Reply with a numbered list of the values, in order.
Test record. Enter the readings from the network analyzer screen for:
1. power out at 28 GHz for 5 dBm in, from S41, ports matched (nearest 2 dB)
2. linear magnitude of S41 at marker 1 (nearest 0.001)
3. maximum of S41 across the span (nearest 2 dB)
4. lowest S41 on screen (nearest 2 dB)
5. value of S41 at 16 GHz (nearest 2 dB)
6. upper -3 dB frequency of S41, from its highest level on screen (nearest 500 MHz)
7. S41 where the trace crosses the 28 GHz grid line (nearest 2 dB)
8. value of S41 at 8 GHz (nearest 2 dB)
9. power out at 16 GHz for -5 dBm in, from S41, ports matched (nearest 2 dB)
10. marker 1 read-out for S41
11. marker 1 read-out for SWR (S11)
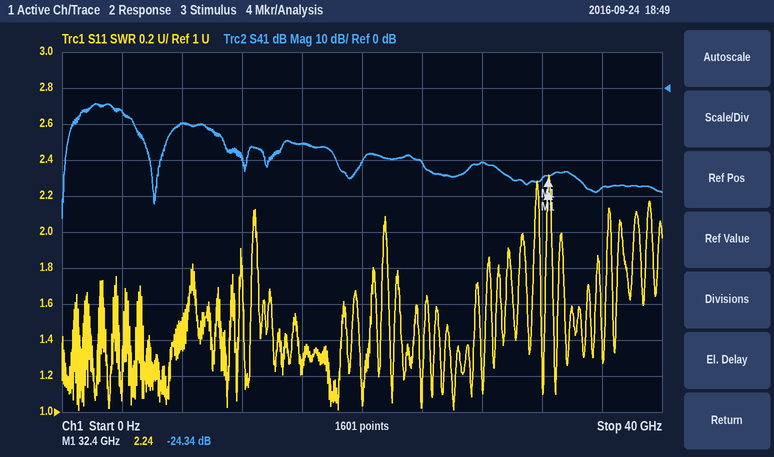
1. -16 dBm
2. 0.061
3. -4 dB
4. -36 dB
5. -16 dB
6. 4.0 GHz
7. -20 dB
8. -10 dB
9. -20 dBm
10. -24.34 dB
11. 2.24
